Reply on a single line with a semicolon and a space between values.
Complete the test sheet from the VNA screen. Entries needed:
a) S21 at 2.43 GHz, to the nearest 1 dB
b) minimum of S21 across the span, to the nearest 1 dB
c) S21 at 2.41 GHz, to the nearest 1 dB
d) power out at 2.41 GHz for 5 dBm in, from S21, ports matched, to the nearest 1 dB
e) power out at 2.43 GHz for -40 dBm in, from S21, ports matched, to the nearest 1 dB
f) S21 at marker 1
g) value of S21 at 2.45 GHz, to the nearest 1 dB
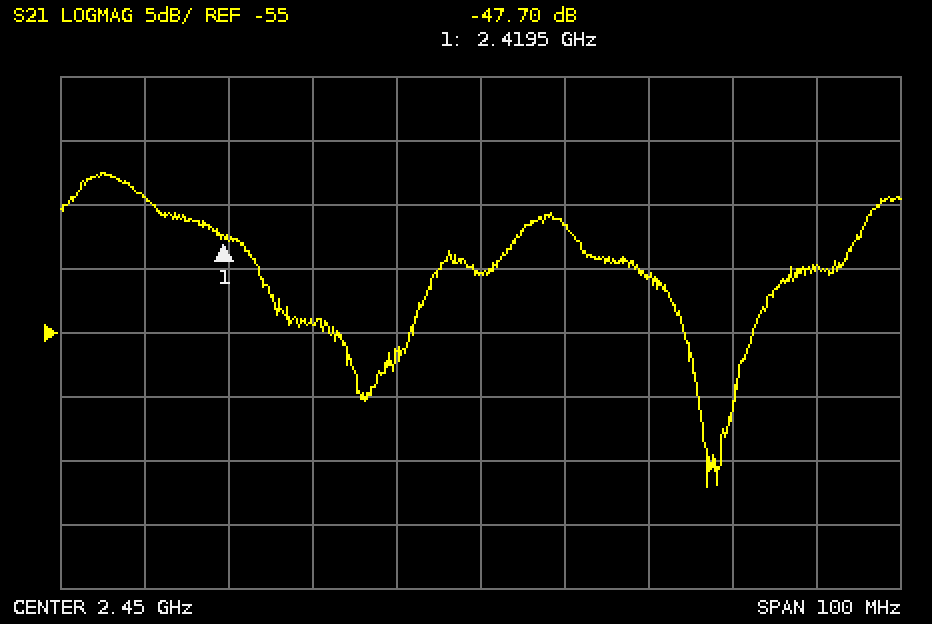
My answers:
-54 dB; -67 dB; -44 dB; -39 dBm; -94 dBm; -47.70 dB; -50 dB
